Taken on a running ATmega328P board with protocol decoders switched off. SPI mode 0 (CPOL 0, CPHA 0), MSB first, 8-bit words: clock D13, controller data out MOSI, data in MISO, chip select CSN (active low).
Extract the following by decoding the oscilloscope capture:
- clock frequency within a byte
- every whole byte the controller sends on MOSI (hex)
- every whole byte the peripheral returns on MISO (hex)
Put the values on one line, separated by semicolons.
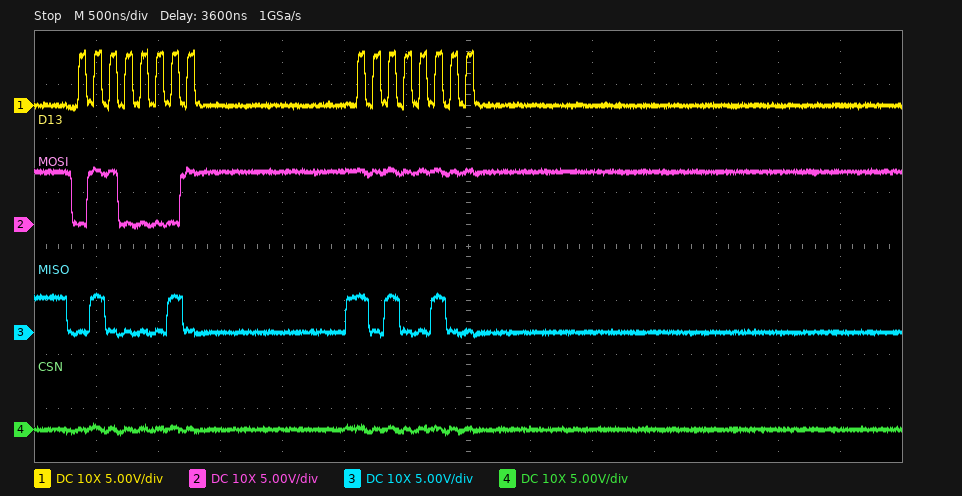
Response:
8 MHz; 61 FF; 42 A4
